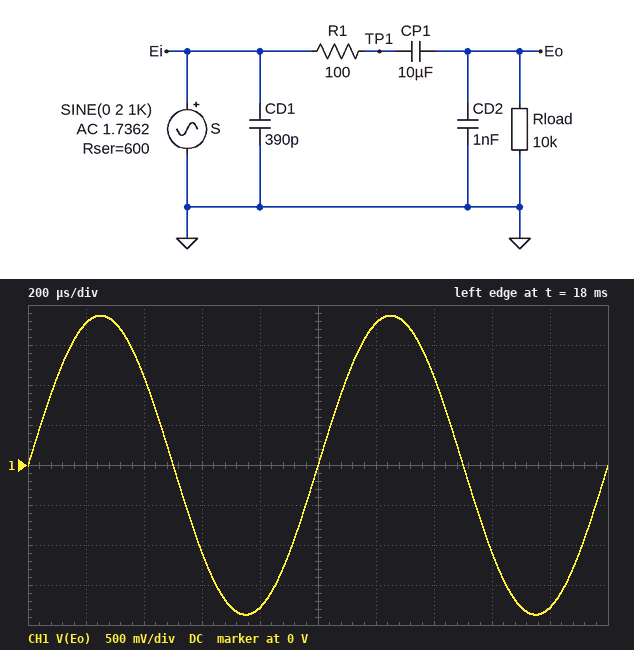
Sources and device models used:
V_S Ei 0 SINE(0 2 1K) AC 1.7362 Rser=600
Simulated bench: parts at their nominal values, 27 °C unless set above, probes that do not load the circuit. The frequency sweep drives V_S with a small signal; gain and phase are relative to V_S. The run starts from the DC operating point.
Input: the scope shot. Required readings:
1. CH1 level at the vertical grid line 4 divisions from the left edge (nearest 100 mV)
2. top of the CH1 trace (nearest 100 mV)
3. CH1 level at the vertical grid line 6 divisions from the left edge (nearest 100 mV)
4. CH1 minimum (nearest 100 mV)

-1.8 V
1.9 V
1.8 V
-1.9 V
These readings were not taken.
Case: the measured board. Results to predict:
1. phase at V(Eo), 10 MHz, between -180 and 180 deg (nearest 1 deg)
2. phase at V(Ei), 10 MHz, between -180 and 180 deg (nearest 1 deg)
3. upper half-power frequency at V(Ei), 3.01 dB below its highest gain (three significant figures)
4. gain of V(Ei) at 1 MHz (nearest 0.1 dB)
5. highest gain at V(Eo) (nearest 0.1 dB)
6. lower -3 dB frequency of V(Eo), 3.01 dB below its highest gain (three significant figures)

-147 deg
-66 deg
168 kHz
-13.9 dB
-0.6 dB
1.49 Hz
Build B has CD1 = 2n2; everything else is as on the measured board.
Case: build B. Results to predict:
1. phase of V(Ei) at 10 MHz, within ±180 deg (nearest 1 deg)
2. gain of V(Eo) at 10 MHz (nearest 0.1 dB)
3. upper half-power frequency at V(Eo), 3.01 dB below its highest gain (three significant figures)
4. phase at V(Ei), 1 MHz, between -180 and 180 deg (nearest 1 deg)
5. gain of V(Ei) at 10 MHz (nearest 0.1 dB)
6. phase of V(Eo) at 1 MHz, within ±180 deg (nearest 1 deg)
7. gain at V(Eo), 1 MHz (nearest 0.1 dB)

-85 deg
-54.6 dB
86.7 kHz
-76 deg
-38.5 dB
-108 deg
-22.6 dB
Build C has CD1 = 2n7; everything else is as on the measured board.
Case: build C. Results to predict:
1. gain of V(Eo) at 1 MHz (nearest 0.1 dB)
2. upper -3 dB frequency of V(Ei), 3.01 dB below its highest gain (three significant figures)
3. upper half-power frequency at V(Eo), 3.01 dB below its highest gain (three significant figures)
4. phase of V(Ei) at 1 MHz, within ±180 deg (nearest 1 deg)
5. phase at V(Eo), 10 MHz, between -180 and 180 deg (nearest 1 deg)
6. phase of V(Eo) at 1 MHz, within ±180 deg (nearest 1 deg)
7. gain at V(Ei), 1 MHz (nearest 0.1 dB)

-23.9 dB
66.7 kHz
75.3 kHz
-78 deg
-167 deg
-110 deg
-22.4 dB
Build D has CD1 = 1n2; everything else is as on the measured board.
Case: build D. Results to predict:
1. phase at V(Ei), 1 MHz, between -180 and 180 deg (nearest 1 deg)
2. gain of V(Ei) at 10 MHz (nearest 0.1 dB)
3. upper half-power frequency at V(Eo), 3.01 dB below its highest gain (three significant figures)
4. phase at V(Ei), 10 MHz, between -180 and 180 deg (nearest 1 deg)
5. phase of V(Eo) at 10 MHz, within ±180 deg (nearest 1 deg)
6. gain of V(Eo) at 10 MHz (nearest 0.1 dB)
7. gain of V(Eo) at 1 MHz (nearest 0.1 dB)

-69 deg
-33.4 dB
124 kHz
-82 deg
-162 deg
-49.5 dB
-19.2 dB
